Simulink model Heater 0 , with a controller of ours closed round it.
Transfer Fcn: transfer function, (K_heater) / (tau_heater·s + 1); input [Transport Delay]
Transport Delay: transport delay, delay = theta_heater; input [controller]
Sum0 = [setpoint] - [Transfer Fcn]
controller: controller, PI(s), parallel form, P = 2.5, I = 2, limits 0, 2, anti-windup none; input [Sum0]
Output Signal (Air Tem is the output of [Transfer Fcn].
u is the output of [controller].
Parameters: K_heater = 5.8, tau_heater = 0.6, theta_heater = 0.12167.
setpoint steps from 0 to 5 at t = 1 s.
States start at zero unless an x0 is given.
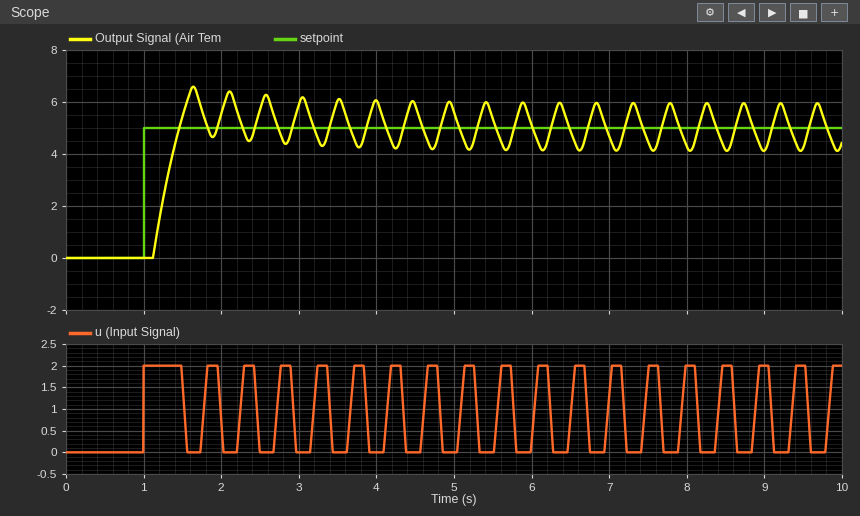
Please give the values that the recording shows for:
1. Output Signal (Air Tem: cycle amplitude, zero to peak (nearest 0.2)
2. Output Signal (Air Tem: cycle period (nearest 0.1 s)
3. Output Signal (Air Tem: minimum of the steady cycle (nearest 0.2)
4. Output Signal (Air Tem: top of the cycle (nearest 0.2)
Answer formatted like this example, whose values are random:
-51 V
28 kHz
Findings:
1.0
0.5 s
4.2
6.0
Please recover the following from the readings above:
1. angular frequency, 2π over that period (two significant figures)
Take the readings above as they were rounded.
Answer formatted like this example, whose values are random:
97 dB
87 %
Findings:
13 rad/s
